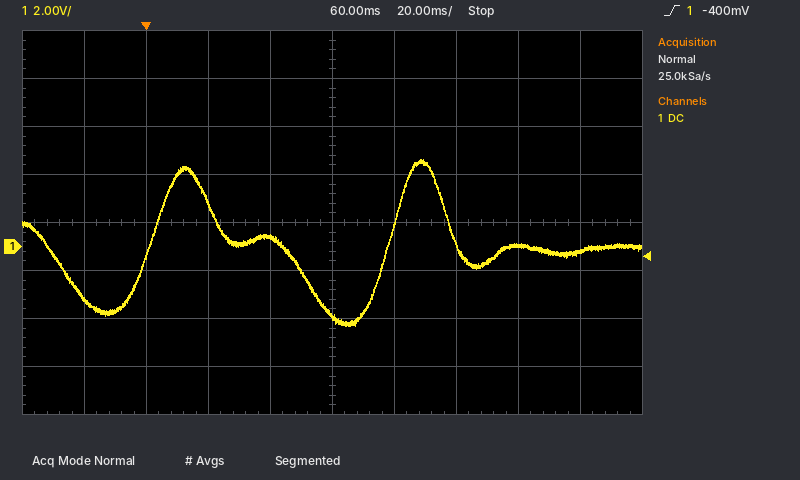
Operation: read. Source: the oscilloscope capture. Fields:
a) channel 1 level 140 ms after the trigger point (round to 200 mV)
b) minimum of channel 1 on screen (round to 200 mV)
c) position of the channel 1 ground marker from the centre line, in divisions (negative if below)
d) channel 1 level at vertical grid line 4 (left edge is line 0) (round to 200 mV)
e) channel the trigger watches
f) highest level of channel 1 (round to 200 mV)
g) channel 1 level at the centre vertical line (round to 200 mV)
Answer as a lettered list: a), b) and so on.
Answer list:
a) -200 mV
b) -3.2 V
c) -0.5 div
d) 400 mV
e) channel 1
f) 3.6 V
g) -2.8 V
